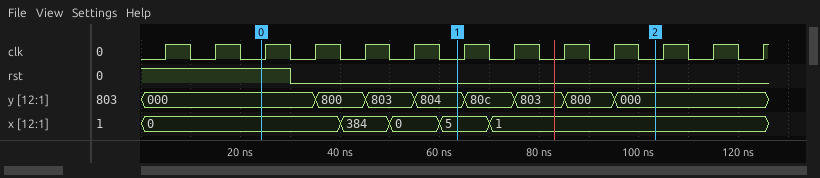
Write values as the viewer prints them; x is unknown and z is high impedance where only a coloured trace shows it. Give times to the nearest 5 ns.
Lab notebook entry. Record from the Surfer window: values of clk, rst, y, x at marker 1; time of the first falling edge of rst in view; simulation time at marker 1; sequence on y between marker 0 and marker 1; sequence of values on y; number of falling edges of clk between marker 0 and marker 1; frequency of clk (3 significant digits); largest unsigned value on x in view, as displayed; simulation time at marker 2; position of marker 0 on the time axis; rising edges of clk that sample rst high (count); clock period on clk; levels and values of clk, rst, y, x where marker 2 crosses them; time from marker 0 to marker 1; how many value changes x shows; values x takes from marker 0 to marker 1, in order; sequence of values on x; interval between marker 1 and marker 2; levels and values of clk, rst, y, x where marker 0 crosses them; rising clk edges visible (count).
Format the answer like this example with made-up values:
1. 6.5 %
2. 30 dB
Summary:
1. clk=0, rst=0, y=804, x=5
2. 30 ns
3. 65 ns
4. 000, 800, 803, 804
5. 000, 800, 803, 804, 80c, 803, 800, 000
6. 4
7. 100 MHz
8. 384
9. 105 ns
10. 25 ns
11. 3
12. 10 ns
13. clk=0, rst=0, y=000, x=1
14. 40 ns
15. 4
16. 0, 384, 0, 5
17. 0, 384, 0, 5, 1
18. 40 ns
19. clk=0, rst=1, y=000, x=0
20. 13
